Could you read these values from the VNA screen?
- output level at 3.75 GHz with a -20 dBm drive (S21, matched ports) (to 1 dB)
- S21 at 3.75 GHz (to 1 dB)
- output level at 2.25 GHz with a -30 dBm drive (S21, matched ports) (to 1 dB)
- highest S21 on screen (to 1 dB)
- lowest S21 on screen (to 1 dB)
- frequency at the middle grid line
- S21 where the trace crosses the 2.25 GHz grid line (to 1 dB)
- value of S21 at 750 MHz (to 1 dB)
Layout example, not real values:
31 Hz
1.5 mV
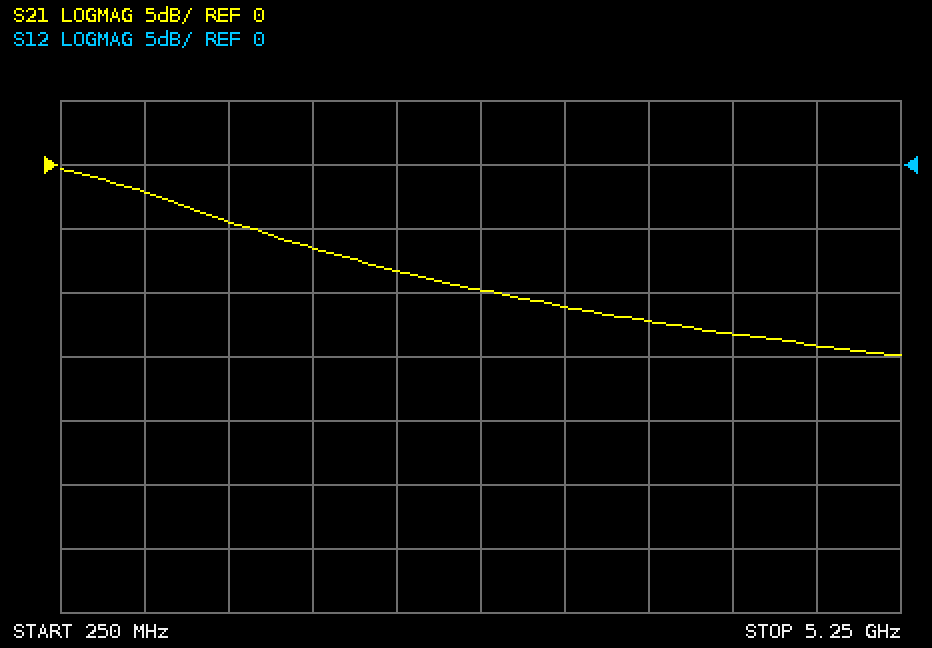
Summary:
-32 dBm
-12 dB
-38 dBm
0 dB
-15 dB
2.75 GHz
-8 dB
-2 dB
